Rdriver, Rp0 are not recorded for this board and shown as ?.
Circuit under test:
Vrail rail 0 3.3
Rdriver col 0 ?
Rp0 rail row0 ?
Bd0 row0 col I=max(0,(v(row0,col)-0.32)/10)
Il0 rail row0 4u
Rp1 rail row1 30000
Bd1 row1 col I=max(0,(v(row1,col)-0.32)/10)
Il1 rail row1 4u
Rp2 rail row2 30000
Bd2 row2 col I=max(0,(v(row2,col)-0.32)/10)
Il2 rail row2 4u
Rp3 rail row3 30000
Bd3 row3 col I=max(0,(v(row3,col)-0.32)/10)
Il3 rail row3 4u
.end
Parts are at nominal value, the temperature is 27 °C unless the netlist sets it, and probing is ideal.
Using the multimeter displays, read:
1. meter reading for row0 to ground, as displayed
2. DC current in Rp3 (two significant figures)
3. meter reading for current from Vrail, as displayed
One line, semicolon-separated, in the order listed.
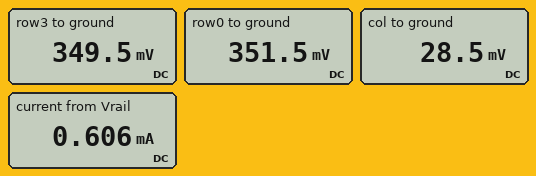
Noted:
351.5 mV; 98 µA; 0.606 mA
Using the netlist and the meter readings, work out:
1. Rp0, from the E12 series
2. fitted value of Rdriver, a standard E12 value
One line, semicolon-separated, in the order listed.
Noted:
10 kΩ; 47 Ω
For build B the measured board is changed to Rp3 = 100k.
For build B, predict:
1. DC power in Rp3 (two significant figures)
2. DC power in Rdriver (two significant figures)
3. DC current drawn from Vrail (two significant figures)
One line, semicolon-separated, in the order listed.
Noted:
87 µW; 14 µW; 540 µA
